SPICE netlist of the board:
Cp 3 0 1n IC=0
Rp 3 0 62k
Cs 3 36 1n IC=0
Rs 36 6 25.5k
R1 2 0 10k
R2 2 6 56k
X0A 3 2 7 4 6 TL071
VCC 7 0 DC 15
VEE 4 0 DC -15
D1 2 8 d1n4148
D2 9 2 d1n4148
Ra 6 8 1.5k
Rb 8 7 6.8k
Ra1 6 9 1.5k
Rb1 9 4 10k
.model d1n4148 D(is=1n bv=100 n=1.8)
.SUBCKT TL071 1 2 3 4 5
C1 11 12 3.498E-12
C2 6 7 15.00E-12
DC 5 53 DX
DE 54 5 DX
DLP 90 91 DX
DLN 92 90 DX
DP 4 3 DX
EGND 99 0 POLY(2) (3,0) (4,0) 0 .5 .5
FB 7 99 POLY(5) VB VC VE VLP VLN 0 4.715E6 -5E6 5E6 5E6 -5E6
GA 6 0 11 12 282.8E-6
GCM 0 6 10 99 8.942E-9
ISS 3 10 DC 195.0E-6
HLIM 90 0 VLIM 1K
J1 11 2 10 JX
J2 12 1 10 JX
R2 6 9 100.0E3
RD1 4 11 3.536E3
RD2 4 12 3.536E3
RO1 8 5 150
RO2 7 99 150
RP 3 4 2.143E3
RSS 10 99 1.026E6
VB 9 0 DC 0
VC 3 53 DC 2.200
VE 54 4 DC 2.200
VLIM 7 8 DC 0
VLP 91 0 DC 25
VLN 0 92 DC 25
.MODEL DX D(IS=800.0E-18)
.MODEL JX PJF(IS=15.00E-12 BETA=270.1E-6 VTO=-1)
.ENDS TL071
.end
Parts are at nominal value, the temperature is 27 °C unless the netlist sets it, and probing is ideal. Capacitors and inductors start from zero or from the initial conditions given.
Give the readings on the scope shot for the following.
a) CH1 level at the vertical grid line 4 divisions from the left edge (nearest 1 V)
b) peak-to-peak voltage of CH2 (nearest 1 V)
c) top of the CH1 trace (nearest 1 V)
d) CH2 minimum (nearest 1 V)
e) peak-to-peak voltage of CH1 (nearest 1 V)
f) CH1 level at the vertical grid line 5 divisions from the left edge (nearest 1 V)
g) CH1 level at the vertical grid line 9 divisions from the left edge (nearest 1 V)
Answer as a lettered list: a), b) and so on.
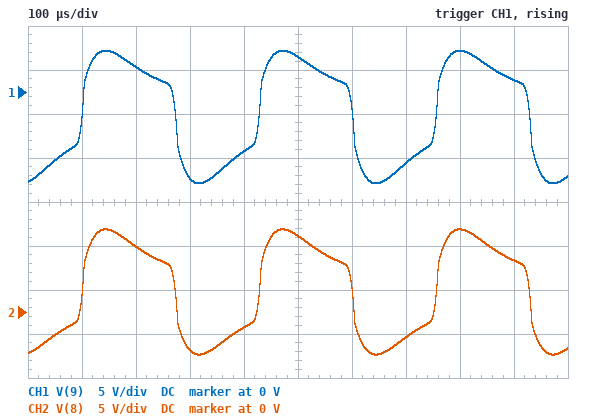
a) -7 V
b) 14 V
c) 5 V
d) -5 V
e) 15 V
f) 4 V
g) 1 V
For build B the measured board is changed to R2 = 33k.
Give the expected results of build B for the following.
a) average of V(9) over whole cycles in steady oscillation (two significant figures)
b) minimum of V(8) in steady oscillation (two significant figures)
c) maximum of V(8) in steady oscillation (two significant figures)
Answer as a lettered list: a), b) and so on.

a) -2.4 V
b) -4.6 V
c) 9.1 V
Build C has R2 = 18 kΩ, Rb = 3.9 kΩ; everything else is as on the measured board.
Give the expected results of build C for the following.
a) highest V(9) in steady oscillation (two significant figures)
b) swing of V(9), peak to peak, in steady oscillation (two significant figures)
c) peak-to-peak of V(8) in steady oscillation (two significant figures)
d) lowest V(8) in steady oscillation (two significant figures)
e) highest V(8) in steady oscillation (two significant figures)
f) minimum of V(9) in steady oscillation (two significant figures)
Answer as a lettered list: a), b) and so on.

a) 5.1 V
b) 19 V
c) 16 V
d) -5.5 V
e) 10 V
f) -14 V
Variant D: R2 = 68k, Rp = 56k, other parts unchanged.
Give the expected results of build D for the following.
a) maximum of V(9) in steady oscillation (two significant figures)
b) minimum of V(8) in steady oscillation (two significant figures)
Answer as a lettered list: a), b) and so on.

a) 4.6 V
b) -4.7 V
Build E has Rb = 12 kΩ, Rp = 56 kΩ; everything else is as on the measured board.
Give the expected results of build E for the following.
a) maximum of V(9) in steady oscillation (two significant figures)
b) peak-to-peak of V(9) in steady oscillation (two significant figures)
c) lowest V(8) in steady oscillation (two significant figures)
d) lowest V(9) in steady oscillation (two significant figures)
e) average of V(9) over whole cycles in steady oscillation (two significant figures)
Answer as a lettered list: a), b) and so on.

a) 3.6 V
b) 11 V
c) -3.6 V
d) -7.4 V
e) -1.9 V
